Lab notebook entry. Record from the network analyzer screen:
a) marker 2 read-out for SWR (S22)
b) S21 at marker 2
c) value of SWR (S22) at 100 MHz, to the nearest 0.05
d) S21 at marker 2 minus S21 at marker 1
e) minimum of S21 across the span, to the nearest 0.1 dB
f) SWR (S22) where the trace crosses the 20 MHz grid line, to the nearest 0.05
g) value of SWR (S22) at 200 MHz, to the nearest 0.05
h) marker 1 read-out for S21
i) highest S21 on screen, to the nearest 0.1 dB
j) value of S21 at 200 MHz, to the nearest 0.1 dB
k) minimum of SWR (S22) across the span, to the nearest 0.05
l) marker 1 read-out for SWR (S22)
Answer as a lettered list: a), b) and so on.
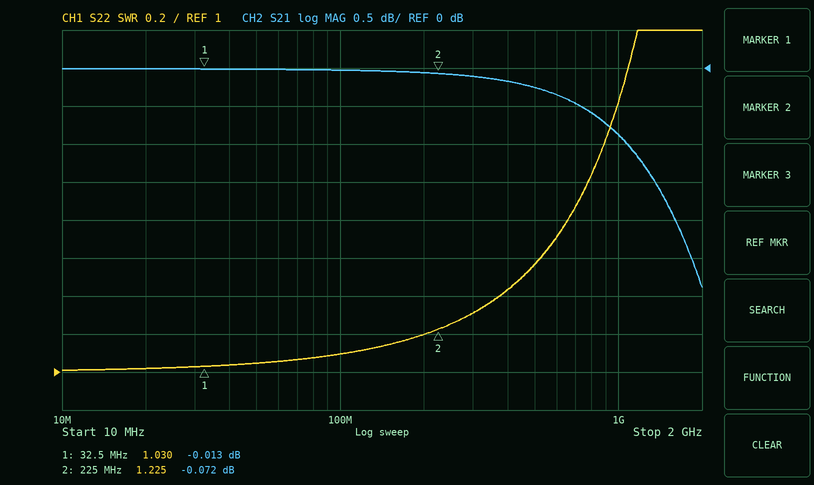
a) 1.225
b) -0.072 dB
c) 1.10
d) -0.059 dB
e) -2.9 dB
f) 1.00
g) 1.20
h) -0.013 dB
i) 0.0 dB
j) -0.1 dB
k) 1.00
l) 1.030
